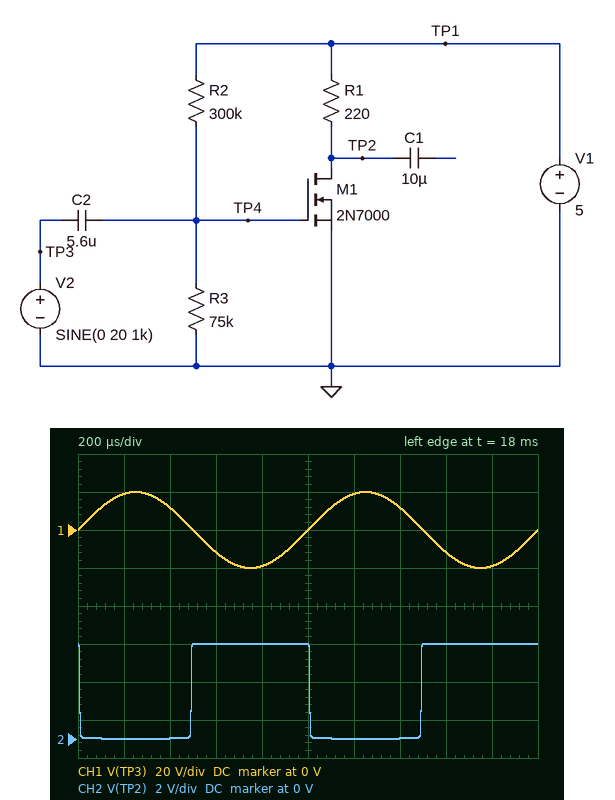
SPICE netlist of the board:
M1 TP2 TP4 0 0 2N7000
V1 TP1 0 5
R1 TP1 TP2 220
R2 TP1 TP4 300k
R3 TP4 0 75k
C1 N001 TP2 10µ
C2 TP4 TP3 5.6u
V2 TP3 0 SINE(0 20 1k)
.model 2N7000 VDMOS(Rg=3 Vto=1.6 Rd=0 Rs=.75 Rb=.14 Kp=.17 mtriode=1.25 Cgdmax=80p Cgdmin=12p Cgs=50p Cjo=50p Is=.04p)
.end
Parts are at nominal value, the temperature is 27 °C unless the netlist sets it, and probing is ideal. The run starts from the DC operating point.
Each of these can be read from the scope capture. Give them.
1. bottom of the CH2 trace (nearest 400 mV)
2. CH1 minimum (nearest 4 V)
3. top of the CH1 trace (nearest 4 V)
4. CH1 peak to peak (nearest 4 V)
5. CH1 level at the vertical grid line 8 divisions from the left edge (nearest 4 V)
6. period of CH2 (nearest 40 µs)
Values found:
0 V
-20 V
20 V
40 V
-12 V
1.00 ms
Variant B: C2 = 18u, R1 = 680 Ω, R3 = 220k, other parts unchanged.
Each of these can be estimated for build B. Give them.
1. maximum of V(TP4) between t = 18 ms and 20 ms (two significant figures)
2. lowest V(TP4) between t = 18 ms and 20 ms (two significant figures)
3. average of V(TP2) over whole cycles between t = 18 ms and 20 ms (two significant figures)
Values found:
22 V
-18 V
2.5 V
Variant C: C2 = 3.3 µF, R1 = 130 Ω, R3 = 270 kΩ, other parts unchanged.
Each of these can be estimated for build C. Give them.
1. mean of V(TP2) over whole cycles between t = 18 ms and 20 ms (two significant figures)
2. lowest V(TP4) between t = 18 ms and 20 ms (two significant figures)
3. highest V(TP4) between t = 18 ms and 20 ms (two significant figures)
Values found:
2.5 V
-18 V
22 V
